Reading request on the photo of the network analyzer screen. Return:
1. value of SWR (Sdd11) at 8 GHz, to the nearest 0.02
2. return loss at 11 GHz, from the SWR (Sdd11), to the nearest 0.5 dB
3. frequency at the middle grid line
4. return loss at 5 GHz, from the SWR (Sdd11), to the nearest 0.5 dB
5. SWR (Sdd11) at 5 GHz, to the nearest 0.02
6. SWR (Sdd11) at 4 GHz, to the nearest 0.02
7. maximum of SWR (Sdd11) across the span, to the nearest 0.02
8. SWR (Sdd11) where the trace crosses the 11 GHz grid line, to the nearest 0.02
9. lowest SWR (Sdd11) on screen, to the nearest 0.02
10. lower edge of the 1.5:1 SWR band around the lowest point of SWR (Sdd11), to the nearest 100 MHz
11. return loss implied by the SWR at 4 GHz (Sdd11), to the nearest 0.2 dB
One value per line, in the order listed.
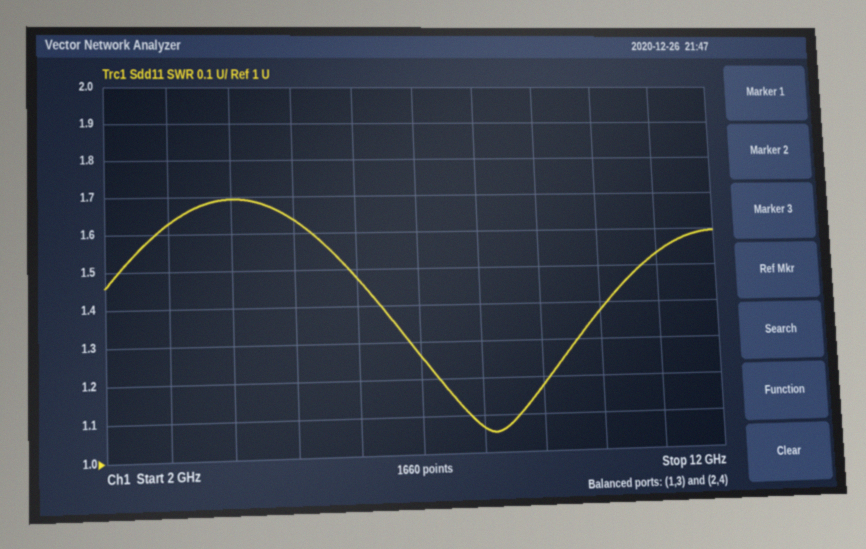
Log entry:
1.06
13.5 dB
7 GHz
12.5 dB
1.64
1.70
1.70
1.54
1.06
5.9 GHz
11.8 dB
